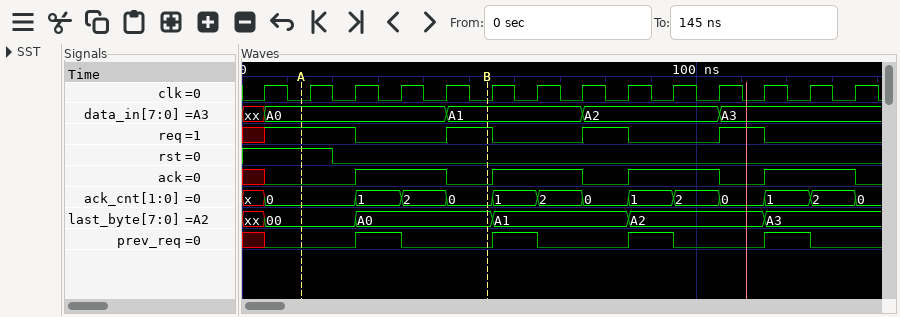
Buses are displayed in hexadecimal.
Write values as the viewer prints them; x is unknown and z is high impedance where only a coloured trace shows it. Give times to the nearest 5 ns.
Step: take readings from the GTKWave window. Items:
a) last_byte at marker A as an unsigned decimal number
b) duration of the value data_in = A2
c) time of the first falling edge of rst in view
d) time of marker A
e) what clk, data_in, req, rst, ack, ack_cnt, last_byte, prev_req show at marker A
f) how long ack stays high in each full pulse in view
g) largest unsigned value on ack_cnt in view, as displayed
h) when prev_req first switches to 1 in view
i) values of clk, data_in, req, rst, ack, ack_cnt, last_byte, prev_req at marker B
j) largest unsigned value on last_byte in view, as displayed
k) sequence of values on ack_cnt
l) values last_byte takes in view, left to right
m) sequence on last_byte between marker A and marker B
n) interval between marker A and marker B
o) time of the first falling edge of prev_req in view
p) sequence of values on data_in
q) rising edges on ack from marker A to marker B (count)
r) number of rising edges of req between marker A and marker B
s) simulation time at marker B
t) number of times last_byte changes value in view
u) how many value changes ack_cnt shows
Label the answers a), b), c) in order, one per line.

a) 0
b) 30 ns
c) 20 ns
d) 15 ns
e) clk=0, data_in=A0, req=1, rst=1, ack=0, ack_cnt=0, last_byte=00, prev_req=0
f) 20 ns, 20 ns, 20 ns, 20 ns
g) 2
h) 25 ns
i) clk=0, data_in=A1, req=1, rst=0, ack=0, ack_cnt=0, last_byte=A0, prev_req=0
j) A3
k) x, 0, 1, 2, 0, 1, 2, 0, 1, 2, 0, 1, 2, 0
l) xx, 00, A0, A1, A2, A3
m) 00, A0
n) 40 ns
o) 35 ns
p) xx, A0, A1, A2, A3
q) 1
r) 1
s) 55 ns
t) 5
u) 13
